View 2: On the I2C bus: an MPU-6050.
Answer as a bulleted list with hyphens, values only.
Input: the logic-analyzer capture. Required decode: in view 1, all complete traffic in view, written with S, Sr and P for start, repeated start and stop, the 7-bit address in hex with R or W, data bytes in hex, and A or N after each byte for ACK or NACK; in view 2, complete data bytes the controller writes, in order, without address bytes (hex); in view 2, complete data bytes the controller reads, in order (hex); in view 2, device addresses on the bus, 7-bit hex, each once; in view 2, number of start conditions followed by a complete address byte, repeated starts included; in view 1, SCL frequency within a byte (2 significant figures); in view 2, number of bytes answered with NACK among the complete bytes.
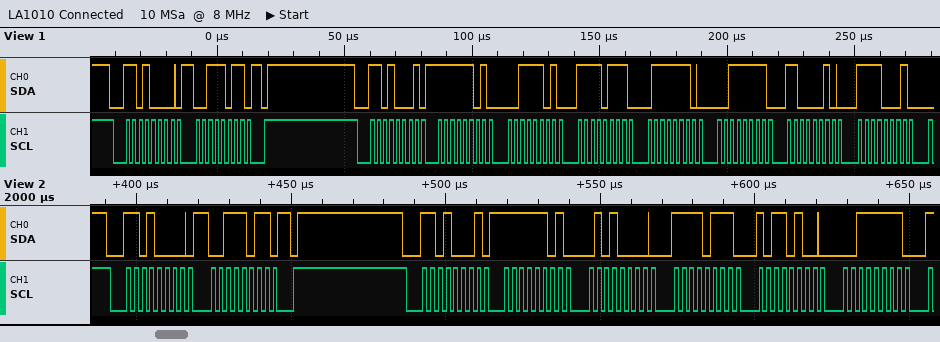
- S 68W A 3B A P S 68R A FD A 3D A F7 A 7E A 3F A C2 A F1 A
- 3B
- FD 50 F7 B4 3F
- 0x68
- 2
- 400 kHz
- 0
